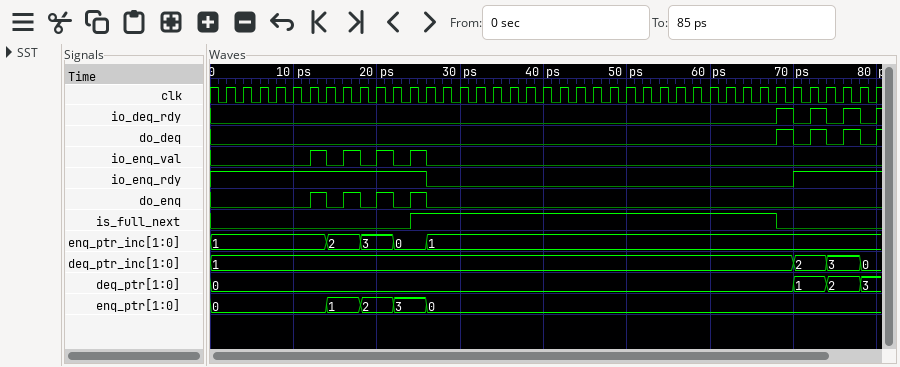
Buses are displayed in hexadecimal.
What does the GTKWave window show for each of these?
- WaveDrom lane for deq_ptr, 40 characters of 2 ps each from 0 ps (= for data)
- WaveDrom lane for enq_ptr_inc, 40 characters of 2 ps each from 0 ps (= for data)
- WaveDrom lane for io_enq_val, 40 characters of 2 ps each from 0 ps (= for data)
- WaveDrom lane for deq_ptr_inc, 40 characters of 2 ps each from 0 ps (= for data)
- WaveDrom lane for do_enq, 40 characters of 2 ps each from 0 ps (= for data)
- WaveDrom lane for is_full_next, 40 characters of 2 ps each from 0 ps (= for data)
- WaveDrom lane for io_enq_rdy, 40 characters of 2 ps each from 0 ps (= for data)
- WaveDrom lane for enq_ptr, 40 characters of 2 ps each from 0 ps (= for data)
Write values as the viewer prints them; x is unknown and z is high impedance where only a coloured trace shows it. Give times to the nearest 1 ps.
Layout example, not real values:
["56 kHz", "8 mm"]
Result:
["{name: 'deq_ptr', wave: '=..................................=.=.=', data: '0 1 2 3'}", "{name: 'enq_ptr_inc', wave: '=......=.=.=.=..........................', data: '1 2 3 0 1'}", "{name: 'io_enq_val', wave: '0.....10101010..........................'}", "{name: 'deq_ptr_inc', wave: '=..................................=.=.=', data: '1 2 3 0'}", "{name: 'do_enq', wave: '0.....10101010..........................'}", "{name: 'is_full_next', wave: '0...........1.....................0.....'}", "{name: 'io_enq_rdy', wave: '1............0.....................1....'}", "{name: 'enq_ptr', wave: '=......=.=.=.=..........................', data: '0 1 2 3 0'}"]
